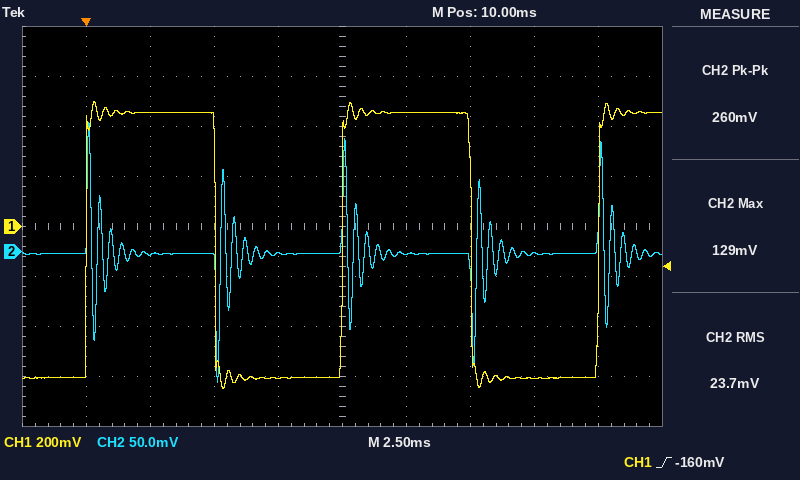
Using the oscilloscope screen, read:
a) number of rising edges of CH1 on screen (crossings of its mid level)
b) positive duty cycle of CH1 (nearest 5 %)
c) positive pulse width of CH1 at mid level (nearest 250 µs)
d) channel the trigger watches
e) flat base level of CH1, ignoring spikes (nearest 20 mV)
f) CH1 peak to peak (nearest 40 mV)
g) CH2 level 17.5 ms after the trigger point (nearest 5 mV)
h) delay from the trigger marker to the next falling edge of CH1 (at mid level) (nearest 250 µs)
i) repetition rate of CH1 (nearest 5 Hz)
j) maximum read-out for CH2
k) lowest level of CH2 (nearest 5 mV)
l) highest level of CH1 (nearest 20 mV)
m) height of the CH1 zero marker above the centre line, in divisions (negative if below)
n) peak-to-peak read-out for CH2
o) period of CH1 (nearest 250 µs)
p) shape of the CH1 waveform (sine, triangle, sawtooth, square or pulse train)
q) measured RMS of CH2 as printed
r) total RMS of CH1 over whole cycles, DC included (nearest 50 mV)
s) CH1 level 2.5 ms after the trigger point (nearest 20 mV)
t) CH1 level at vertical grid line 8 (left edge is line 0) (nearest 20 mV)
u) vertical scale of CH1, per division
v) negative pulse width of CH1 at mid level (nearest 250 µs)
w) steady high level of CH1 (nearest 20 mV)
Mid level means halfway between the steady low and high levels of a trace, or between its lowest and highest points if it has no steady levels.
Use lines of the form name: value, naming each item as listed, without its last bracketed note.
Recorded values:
number of rising edges of CH1 on screen: 3
positive duty cycle of CH1: 50 %
positive pulse width of CH1 at mid level: 5.00 ms
channel the trigger watches: CH1
flat base level of CH1, ignoring spikes: -600 mV
CH1 peak to peak: 1.16 V
CH2 level 17.5 ms after the trigger point: 0 mV
delay from the trigger marker to the next falling edge of CH1 (at mid level): 5.00 ms
repetition rate of CH1: 100 Hz
maximum read-out for CH2: 129 mV
lowest level of CH2: -130 mV
highest level of CH1: 500 mV
height of the CH1 zero marker above the centre line, in divisions: 0.0 div
peak-to-peak read-out for CH2: 260 mV
period of CH1: 10.00 ms
shape of the CH1 waveform: square
measured RMS of CH2 as printed: 23.7 mV
total RMS of CH1 over whole cycles, DC included: 550 mV
CH1 level 2.5 ms after the trigger point: 460 mV
CH1 level at vertical grid line 8 (left edge is line 0): -600 mV
vertical scale of CH1, per division: 200 mV
negative pulse width of CH1 at mid level: 5.00 ms
steady high level of CH1: 460 mV
